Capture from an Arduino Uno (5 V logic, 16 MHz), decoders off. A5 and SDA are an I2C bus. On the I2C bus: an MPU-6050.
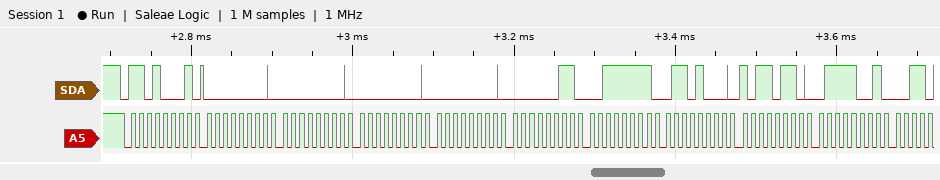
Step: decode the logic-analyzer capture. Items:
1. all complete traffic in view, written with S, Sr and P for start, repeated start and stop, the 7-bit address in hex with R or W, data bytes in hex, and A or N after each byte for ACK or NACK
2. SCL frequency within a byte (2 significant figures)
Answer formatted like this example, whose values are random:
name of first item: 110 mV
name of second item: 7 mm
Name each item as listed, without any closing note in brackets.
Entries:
all complete traffic in view, written with S, Sr and P for start, repeated start and stop, the 7-bit address in hex with R or W, data bytes in hex, and A or N after each byte for ACK or NACK: S 68R A 00 A 00 A 00 A 00 A 03 A 3F A 68 A B6 A 79 A
SCL frequency within a byte: 100 kHz
